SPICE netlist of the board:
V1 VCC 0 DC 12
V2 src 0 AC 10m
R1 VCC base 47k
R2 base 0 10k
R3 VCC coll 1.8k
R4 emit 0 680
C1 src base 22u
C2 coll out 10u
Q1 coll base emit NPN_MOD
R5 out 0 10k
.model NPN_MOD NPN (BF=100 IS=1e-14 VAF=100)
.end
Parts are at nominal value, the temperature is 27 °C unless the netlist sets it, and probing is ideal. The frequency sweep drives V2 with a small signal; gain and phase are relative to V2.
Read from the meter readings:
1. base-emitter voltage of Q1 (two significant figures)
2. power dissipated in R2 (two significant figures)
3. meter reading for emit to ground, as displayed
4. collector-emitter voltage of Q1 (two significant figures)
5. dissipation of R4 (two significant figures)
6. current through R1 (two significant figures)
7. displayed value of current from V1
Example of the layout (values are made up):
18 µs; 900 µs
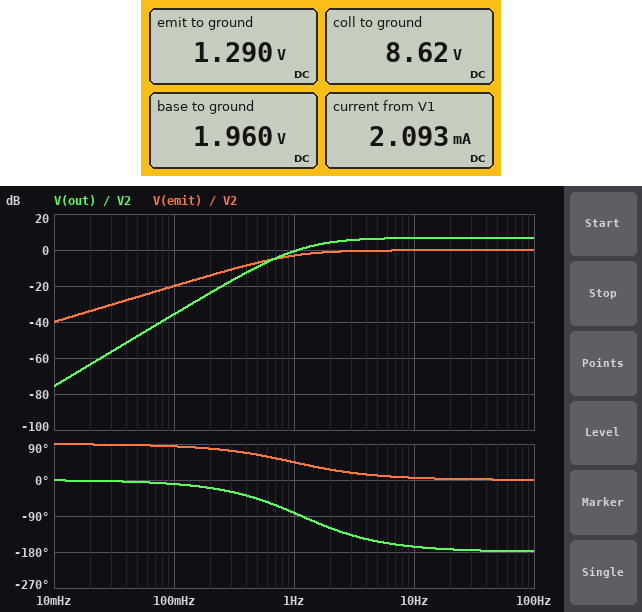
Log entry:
670 mV; 380 µW; 1.290 V; 7.3 V; 2.4 mW; 210 µA; 2.093 mA
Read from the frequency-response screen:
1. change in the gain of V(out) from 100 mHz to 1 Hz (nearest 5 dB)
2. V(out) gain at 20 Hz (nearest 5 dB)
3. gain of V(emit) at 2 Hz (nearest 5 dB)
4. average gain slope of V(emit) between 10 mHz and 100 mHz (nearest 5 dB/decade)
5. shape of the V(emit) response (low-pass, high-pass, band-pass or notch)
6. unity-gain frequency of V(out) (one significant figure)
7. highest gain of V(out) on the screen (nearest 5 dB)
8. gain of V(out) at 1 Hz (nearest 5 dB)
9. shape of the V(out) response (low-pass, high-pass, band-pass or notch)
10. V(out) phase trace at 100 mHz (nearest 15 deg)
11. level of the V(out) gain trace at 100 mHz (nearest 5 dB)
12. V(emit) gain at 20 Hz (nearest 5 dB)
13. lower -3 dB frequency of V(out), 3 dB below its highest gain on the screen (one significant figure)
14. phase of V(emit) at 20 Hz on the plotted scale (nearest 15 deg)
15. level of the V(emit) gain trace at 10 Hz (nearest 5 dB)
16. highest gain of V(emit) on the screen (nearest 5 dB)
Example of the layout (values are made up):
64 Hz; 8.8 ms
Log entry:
35 dB; 5 dB; 0 dB; 20 dB/decade; high-pass; 1 Hz; 5 dB; 0 dB; high-pass; -15 deg; -35 dB; 0 dB; 2 Hz; 0 deg; 0 dB; 0 dB
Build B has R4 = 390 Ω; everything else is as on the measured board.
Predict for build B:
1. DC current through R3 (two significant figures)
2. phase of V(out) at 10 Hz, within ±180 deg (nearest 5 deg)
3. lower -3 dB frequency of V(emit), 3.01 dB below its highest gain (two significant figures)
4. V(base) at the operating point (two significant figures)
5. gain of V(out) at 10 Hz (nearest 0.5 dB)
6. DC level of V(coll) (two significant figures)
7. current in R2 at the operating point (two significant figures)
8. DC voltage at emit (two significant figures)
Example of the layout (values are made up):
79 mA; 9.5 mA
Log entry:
3.0 mA; -165 deg; 1.1 Hz; 1.9 V; 11.5 dB; 6.6 V; 190 µA; 1.2 V
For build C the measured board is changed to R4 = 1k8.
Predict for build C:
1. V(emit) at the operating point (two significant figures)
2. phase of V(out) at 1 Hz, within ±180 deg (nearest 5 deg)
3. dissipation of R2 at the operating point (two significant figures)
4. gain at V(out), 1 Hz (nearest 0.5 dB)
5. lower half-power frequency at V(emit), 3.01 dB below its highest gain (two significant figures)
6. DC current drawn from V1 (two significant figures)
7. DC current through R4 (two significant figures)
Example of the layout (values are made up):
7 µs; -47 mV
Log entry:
1.4 V; -85 deg; 420 µW; -9.0 dB; 910 mHz; 980 µA; 780 µA
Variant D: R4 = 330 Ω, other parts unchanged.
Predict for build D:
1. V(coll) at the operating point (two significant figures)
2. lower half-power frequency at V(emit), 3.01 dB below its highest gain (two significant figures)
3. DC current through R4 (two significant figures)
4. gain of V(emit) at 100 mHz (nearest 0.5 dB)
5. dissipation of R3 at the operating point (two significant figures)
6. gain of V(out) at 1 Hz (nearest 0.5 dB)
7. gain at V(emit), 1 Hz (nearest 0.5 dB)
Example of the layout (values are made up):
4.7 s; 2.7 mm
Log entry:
5.8 V; 1.1 Hz; 3.5 mA; -21.0 dB; 21 mW; 5.0 dB; -3.5 dB
